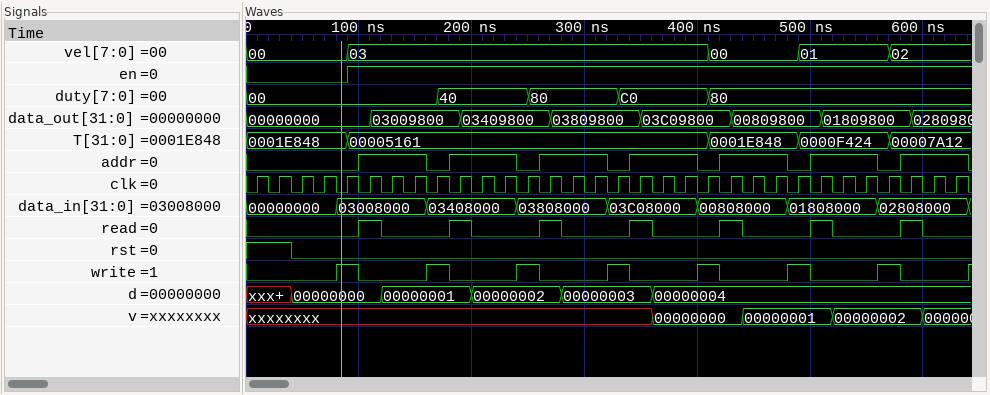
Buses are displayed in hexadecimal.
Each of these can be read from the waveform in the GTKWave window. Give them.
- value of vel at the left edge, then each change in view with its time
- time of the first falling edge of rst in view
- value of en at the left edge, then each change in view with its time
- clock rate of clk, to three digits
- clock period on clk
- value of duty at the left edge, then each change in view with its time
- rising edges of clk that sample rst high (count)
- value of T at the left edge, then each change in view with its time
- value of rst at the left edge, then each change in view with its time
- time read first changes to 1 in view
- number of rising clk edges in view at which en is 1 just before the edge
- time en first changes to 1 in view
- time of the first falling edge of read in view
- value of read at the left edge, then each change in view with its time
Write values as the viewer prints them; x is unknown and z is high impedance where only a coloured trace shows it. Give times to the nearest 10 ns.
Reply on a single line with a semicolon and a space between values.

00, 03 at 90 ns, 00 at 410 ns, 01 at 490 ns, 02 at 570 ns; 40 ns; 0, 1 at 90 ns; 50.0 MHz; 20 ns; 00, 40 at 170 ns, 80 at 250 ns, C0 at 330 ns, 80 at 410 ns; 2; 0001E848, 00005161 at 90 ns, 0001E848 at 410 ns, 0000F424 at 490 ns, 00007A12 at 570 ns; 1, 0 at 40 ns; 100 ns; 27; 90 ns; 120 ns; 0, 1 at 100 ns, 0 at 120 ns, 1 at 180 ns, 0 at 200 ns, 1 at 260 ns, 0 at 280 ns, 1 at 340 ns, 0 at 360 ns, 1 at 420 ns, 0 at 440 ns, 1 at 500 ns, 0 at 520 ns, 1 at 580 ns, 0 at 600 ns
